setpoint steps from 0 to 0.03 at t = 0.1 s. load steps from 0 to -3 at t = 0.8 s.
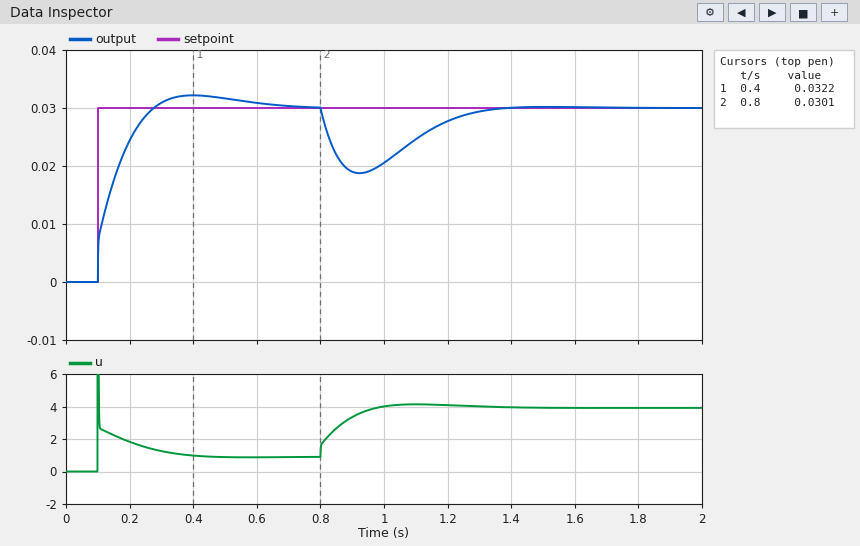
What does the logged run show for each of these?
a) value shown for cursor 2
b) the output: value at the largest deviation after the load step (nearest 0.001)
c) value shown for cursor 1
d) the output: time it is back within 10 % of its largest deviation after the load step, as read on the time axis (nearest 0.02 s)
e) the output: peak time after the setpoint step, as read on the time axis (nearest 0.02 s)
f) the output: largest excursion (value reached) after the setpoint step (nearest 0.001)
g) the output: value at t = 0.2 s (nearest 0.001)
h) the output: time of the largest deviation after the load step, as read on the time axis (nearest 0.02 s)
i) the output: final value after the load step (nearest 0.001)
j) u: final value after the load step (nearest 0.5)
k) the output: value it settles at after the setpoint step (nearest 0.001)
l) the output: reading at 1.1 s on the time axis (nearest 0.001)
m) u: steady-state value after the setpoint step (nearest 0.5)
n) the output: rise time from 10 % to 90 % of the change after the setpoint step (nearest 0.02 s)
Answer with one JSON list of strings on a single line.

["0.0301", "0.019", "0.0322", "1.26 s", "0.40 s", "0.032", "0.024", "0.92 s", "0.030", "4.0", "0.030", "0.025", "1.0", "0.12 s"]
